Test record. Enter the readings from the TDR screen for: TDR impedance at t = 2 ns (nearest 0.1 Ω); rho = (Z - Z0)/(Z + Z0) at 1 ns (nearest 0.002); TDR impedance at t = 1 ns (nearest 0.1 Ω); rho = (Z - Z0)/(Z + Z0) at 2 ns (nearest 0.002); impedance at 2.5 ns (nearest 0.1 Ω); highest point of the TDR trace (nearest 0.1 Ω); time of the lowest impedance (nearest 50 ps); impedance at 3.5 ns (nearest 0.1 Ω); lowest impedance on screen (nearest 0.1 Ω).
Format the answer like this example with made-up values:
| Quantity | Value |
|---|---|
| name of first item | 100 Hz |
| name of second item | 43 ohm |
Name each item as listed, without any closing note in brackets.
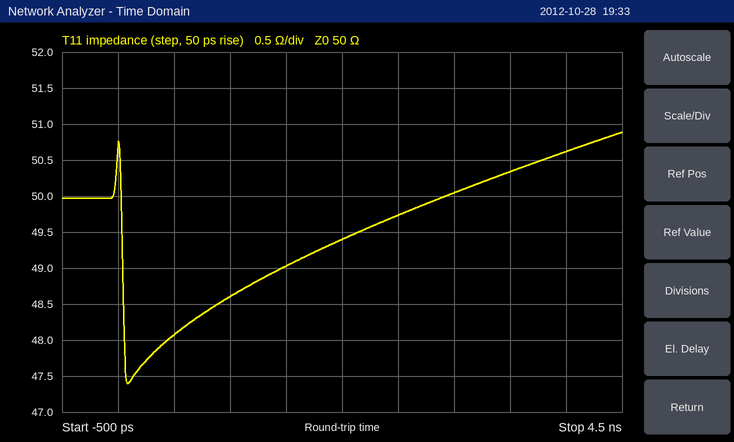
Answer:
| Quantity | Value |
|---|---|
| TDR impedance at t = 2 ns | 49.4 Ω |
| rho = (Z - Z0)/(Z + Z0) at 1 ns | -0.014 |
| TDR impedance at t = 1 ns | 48.6 Ω |
| rho = (Z - Z0)/(Z + Z0) at 2 ns | -0.006 |
| impedance at 2.5 ns | 49.7 Ω |
| highest point of the TDR trace | 50.9 Ω |
| time of the lowest impedance | 100 ps |
| impedance at 3.5 ns | 50.3 Ω |
| lowest impedance on screen | 47.4 Ω |
